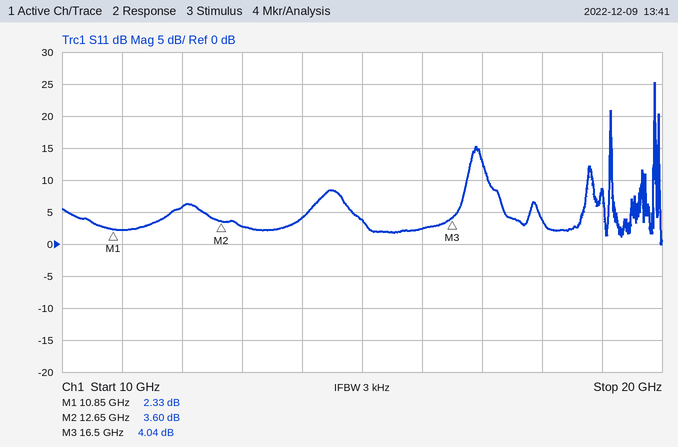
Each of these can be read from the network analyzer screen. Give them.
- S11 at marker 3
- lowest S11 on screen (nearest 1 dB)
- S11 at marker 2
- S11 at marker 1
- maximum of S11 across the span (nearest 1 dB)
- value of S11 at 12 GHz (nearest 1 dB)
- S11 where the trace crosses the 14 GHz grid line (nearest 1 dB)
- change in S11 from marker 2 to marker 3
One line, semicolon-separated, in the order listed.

4.04 dB; 0 dB; 3.60 dB; 2.33 dB; 25 dB; 6 dB; 4 dB; 0.44 dB
